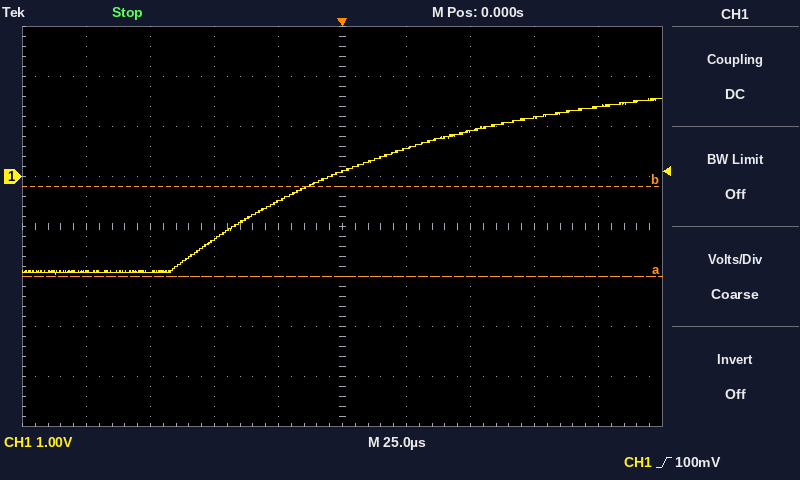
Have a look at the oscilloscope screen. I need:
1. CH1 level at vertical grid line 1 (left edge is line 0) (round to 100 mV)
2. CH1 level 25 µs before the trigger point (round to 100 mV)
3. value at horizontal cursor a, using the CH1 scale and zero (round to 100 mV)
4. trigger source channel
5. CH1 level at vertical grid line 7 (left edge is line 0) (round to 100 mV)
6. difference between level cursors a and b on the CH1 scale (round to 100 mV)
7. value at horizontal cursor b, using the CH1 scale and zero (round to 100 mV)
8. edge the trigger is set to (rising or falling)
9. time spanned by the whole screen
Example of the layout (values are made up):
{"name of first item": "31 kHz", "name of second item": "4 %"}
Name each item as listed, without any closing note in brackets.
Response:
{"CH1 level at vertical grid line 1 (left edge is line 0)": "-1.9 V", "CH1 level 25 µs before the trigger point": "-500 mV", "value at horizontal cursor a, using the CH1 scale and zero": "-2.0 V", "trigger source channel": "CH1", "CH1 level at vertical grid line 7 (left edge is line 0)": "900 mV", "difference between level cursors a and b on the CH1 scale": "1.8 V", "value at horizontal cursor b, using the CH1 scale and zero": "-200 mV", "edge the trigger is set to": "rising", "time spanned by the whole screen": "250 µs"}
